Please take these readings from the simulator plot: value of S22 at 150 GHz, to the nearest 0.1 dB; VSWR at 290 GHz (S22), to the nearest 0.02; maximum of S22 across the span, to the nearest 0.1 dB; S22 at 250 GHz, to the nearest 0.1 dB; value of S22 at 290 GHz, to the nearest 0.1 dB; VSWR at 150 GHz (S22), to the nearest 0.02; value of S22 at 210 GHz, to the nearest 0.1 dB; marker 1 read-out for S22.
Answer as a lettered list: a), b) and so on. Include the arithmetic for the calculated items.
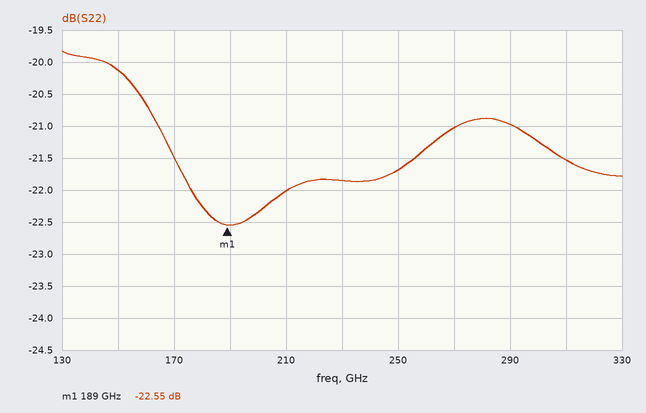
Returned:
a) -20.1 dB
b) |Γ| = 10^(-21/20) = 0.0891; VSWR = (1 + 0.0891)/(1 − 0.0891) ≈ 1.20
c) -19.8 dB
d) -21.7 dB
e) -21.0 dB
f) |Γ| = 10^(-20.1/20) = 0.0989; VSWR = (1 + 0.0989)/(1 − 0.0989) ≈ 1.22
g) -22.0 dB
h) -22.55 dB
